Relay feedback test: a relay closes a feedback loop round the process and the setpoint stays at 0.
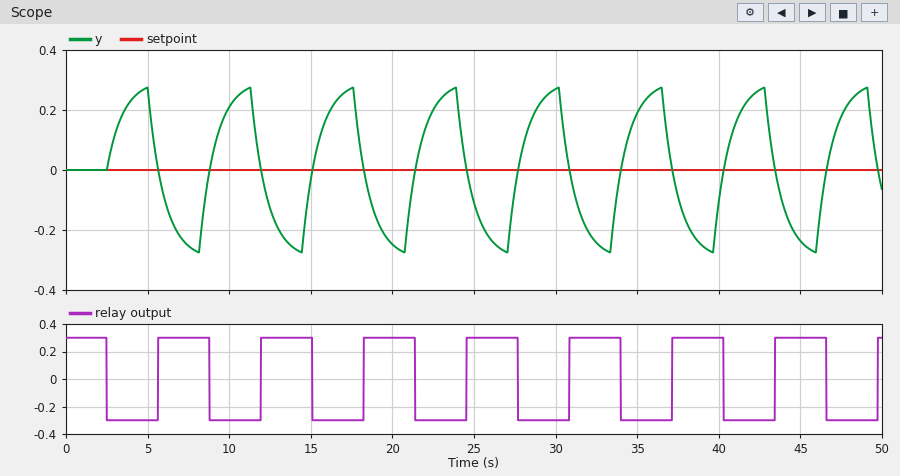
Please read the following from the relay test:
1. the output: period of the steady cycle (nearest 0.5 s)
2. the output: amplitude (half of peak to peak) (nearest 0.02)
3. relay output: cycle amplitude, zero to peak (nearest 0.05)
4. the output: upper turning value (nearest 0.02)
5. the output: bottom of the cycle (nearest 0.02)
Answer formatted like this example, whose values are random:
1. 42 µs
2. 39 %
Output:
1. 6.5 s
2. 0.28
3. 0.30
4. 0.28
5. -0.28
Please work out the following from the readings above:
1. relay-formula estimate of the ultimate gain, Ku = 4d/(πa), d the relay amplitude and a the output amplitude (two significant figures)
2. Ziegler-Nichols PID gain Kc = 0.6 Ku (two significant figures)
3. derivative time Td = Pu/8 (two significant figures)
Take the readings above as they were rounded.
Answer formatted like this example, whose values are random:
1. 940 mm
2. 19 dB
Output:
1. 1.4
2. 0.84
3. 0.81 s
